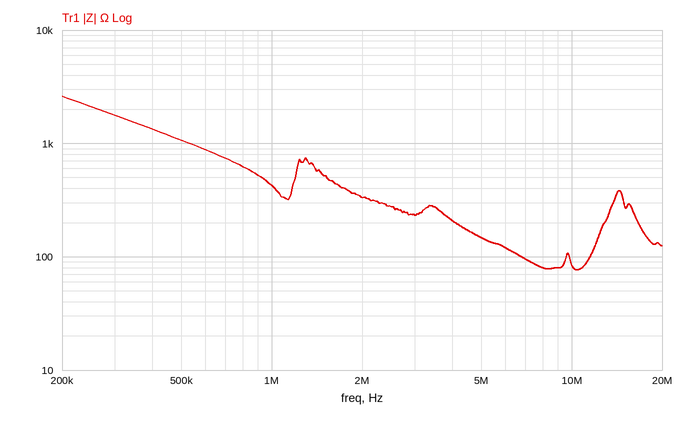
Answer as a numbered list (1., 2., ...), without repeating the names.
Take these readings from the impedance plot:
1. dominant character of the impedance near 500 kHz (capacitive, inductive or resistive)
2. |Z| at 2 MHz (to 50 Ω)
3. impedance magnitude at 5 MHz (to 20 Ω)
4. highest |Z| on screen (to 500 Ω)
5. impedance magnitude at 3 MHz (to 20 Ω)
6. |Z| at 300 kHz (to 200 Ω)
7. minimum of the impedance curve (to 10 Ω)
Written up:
1. capacitive
2. 350 Ω
3. 140 Ω
4. 2.5 kΩ
5. 240 Ω
6. 1.8 kΩ
7. 80 Ω
